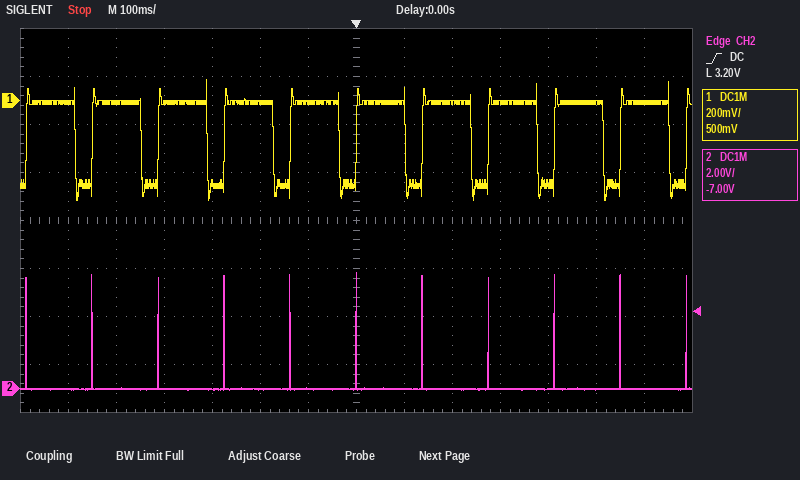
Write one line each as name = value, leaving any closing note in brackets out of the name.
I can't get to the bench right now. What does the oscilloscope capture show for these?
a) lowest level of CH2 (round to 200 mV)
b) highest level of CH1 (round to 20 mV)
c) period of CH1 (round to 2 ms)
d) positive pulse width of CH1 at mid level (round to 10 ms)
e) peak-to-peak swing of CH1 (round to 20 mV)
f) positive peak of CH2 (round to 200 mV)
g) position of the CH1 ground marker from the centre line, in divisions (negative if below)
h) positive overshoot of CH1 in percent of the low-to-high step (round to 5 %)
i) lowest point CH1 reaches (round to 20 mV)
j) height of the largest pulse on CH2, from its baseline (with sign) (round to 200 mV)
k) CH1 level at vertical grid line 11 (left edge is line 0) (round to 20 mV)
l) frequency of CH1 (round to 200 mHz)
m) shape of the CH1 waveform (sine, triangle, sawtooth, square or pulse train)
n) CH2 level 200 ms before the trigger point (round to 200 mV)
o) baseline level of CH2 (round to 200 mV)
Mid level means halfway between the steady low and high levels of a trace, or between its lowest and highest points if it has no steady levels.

lowest level of CH2 = 0.0 V
highest level of CH1 = 80 mV
period of CH1 = 138 ms
positive pulse width of CH1 at mid level = 100 ms
peak-to-peak swing of CH1 = 500 mV
positive peak of CH2 = 4.8 V
position of the CH1 ground marker from the centre line, in divisions = +2.5 div
positive overshoot of CH1 in percent of the low-to-high step = 30 %
lowest point CH1 reaches = -420 mV
height of the largest pulse on CH2, from its baseline (with sign) = +4.8 V
CH1 level at vertical grid line 11 (left edge is line 0) = -340 mV
frequency of CH1 = 7.2 Hz
shape of the CH1 waveform = pulse train
CH2 level 200 ms before the trigger point = 0.0 V
baseline level of CH2 = 0.0 V
